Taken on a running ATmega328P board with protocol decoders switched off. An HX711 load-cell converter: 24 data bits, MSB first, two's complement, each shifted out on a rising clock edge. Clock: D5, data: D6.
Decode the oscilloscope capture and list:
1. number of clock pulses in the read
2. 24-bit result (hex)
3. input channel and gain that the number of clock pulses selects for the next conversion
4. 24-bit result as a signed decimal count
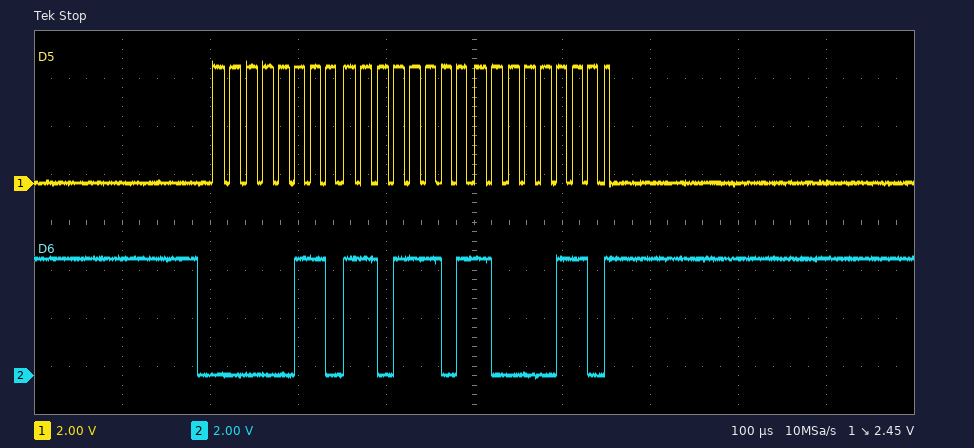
25
0x06DD86
channel A, gain 128
449926
